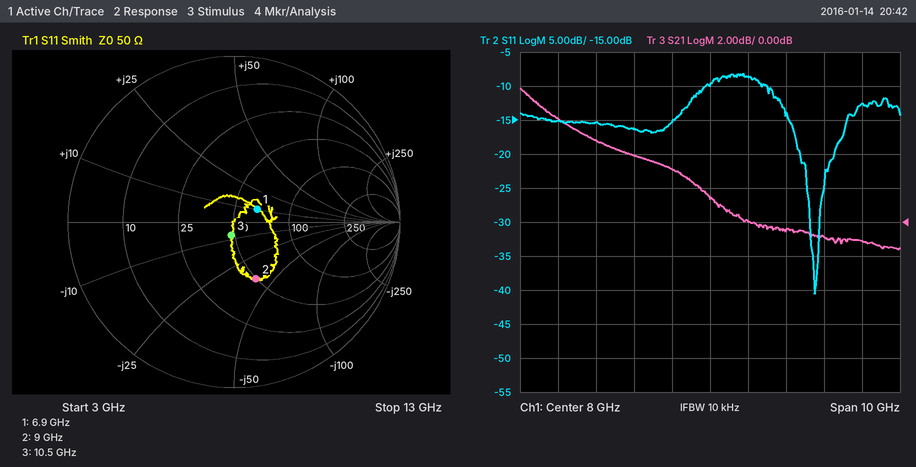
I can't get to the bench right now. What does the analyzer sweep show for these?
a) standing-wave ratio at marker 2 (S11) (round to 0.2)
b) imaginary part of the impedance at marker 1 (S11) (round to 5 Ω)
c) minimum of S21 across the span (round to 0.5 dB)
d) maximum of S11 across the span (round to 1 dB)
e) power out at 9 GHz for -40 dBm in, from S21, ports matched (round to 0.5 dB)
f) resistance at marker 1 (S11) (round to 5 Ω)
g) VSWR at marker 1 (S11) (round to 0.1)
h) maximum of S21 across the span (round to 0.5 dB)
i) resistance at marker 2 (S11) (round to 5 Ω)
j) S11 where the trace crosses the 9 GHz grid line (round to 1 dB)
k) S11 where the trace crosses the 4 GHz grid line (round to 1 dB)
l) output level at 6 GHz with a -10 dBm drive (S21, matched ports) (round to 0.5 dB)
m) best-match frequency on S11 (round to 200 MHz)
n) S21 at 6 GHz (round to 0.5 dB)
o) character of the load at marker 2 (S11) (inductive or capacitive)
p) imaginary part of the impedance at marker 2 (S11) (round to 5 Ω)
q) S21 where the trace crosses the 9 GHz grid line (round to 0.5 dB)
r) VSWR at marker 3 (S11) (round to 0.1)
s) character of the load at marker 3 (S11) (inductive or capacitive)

2.2
+10 Ω
-1.5 dB
-8 dB
-40.0 dBm
65 Ω
1.4
8.0 dB
50 Ω
-9 dB
-15 dB
-6.0 dBm
10.8 GHz
4.0 dB
capacitive
-40 Ω
0.0 dB
1.2
capacitive
